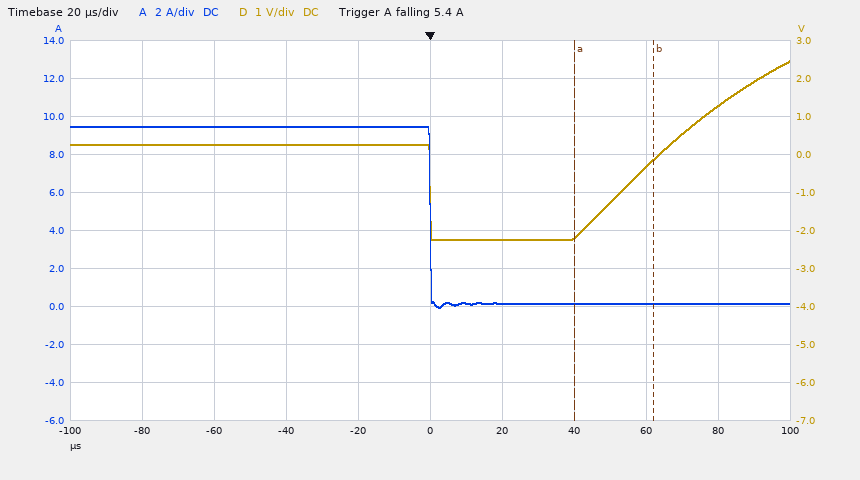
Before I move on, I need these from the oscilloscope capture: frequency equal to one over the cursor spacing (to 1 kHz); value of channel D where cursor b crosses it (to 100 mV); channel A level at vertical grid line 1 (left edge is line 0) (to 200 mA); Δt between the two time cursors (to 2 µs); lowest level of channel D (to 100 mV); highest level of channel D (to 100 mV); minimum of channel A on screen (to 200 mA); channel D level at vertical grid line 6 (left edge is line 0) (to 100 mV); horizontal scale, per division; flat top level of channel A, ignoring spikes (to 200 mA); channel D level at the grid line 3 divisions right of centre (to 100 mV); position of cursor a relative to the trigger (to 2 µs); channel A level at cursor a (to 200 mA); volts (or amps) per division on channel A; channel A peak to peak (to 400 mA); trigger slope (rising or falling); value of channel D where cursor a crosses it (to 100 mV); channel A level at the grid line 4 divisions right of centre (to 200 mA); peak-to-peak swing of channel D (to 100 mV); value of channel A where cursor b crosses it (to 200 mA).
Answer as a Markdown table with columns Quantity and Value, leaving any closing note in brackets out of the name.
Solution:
| Quantity | Value |
|---|---|
| frequency equal to one over the cursor spacing | 45 kHz |
| value of channel D where cursor b crosses it | -100 mV |
| channel A level at vertical grid line 1 (left edge is line 0) | 9.4 A |
| Δt between the two time cursors | 22 µs |
| lowest level of channel D | -2.2 V |
| highest level of channel D | 2.5 V |
| minimum of channel A on screen | 0.0 A |
| channel D level at vertical grid line 6 (left edge is line 0) | -2.2 V |
| horizontal scale, per division | 20 µs |
| flat top level of channel A, ignoring spikes | 9.4 A |
| channel D level at the grid line 3 divisions right of centre | -300 mV |
| position of cursor a relative to the trigger | +40 µs |
| channel A level at cursor a | 200 mA |
| volts (or amps) per division on channel A | 2 A |
| channel A peak to peak | 9.6 A |
| trigger slope | falling |
| value of channel D where cursor a crosses it | -2.2 V |
| channel A level at the grid line 4 divisions right of centre | 200 mA |
| peak-to-peak swing of channel D | 4.7 V |
| value of channel A where cursor b crosses it | 200 mA |
